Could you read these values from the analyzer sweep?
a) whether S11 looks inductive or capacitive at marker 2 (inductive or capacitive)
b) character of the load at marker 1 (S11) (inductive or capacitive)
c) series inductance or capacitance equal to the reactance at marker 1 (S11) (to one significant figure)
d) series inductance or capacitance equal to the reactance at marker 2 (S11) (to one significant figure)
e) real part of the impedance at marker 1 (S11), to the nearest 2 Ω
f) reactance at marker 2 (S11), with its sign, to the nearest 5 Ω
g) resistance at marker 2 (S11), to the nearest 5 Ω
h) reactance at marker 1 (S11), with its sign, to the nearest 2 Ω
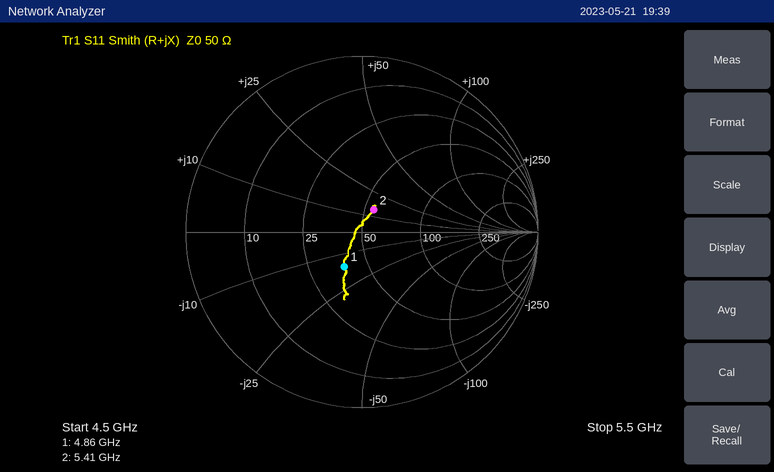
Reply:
inductive
capacitive
2 pF
400 pH
38 Ω
+15 Ω
55 Ω
-16 Ω
